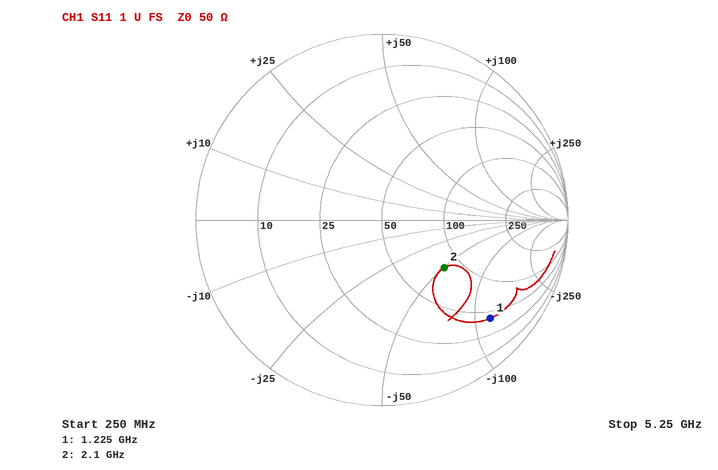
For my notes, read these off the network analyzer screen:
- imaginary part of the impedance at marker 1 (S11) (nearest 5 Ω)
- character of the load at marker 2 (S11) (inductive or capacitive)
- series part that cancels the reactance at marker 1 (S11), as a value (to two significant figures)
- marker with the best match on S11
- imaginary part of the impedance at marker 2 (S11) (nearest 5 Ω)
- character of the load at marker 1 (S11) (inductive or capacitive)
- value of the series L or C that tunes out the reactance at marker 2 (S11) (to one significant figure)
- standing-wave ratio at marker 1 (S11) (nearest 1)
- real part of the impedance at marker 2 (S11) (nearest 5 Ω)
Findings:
-115 Ω
capacitive
15 nH
marker 2
-50 Ω
capacitive
4 nH
8
80 Ω
